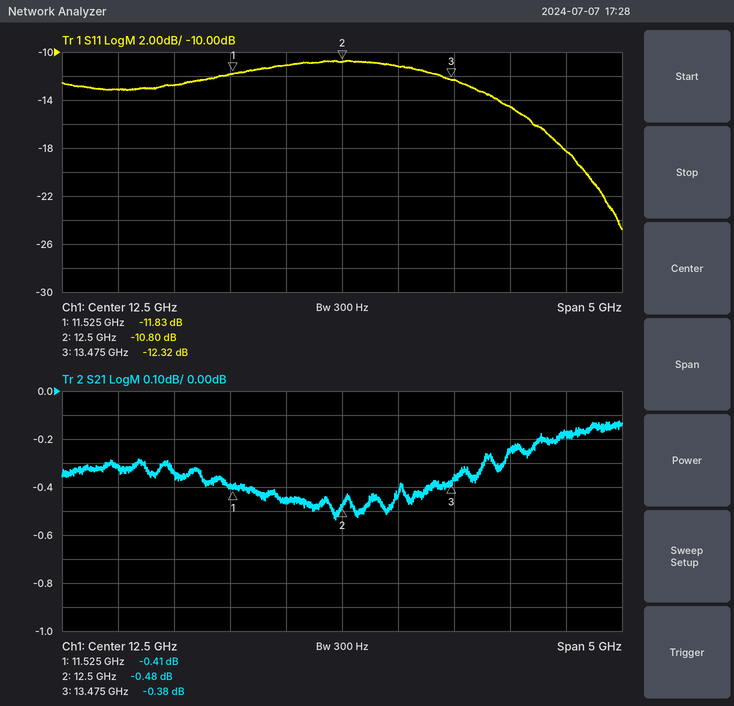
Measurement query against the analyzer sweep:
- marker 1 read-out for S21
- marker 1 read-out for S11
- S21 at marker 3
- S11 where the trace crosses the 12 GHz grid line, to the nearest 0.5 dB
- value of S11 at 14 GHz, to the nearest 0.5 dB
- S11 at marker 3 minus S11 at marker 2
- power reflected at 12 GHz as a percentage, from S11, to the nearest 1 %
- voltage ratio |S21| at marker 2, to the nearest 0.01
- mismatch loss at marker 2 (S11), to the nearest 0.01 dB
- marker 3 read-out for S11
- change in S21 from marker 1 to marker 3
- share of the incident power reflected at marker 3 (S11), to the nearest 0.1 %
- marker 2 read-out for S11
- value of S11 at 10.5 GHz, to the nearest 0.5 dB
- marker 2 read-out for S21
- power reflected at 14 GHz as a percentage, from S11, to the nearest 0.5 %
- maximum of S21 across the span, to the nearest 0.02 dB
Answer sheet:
-0.41 dB
-11.83 dB
-0.38 dB
-11.0 dB
-14.5 dB
-1.52 dB
8 %
0.95
0.38 dB
-12.32 dB
0.03 dB
5.9 %
-10.80 dB
-13.0 dB
-0.48 dB
3.5 %
-0.12 dB
